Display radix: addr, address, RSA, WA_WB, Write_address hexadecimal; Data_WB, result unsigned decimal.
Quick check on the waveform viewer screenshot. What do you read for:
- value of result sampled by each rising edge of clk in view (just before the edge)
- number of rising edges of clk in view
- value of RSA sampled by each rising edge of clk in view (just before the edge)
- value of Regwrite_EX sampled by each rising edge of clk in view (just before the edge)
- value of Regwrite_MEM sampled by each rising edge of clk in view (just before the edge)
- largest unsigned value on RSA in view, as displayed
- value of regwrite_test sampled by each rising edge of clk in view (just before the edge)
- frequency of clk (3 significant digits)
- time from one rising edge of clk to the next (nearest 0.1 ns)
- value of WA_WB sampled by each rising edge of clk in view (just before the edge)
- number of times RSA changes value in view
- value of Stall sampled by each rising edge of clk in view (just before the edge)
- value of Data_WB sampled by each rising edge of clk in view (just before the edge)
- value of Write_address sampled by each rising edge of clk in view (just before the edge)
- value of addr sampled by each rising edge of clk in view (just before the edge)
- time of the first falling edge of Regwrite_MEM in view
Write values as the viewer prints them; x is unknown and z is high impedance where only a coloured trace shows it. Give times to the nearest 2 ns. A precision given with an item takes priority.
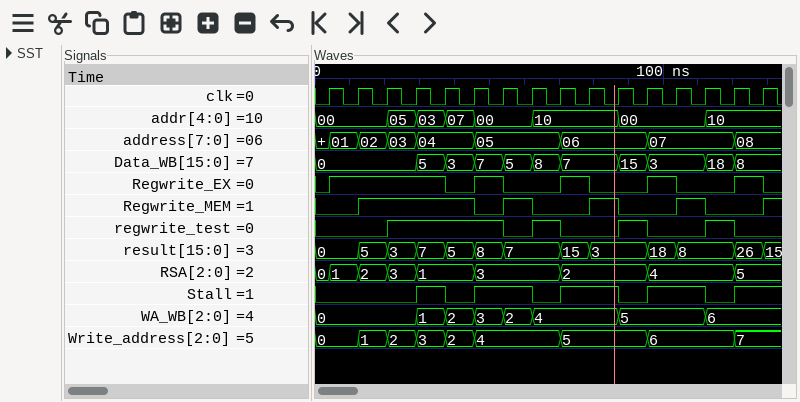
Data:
0, 0, 5, 3, 7, 5, 8, 7, 7, 15, 3, 3, 18, 8, 8, 26
16
0, 1, 2, 3, 1, 1, 3, 3, 3, 2, 2, 2, 4, 4, 4, 5
0 1 1 1 1 0 1 0 0 1 0 0 1 0 0 1
0 0 1 1 1 1 0 1 0 0 1 0 0 1 0 0
5
0 0 0 1 1 1 1 0 1 0 0 1 0 0 1 0
120 MHz
8.3 ns
0, 0, 0, 0, 1, 2, 3, 2, 4, 4, 4, 5, 5, 5, 6, 6
8
0 0 0 0 1 0 1 1 0 1 1 0 1 1 0 1
0, 0, 0, 0, 5, 3, 7, 5, 8, 7, 7, 15, 3, 3, 18, 8
0, 0, 1, 2, 3, 2, 4, 4, 4, 5, 5, 5, 6, 6, 6, 7
00, 00, 00, 05, 03, 07, 00, 00, 10, 10, 10, 00, 00, 00, 10, 10
46 ns
